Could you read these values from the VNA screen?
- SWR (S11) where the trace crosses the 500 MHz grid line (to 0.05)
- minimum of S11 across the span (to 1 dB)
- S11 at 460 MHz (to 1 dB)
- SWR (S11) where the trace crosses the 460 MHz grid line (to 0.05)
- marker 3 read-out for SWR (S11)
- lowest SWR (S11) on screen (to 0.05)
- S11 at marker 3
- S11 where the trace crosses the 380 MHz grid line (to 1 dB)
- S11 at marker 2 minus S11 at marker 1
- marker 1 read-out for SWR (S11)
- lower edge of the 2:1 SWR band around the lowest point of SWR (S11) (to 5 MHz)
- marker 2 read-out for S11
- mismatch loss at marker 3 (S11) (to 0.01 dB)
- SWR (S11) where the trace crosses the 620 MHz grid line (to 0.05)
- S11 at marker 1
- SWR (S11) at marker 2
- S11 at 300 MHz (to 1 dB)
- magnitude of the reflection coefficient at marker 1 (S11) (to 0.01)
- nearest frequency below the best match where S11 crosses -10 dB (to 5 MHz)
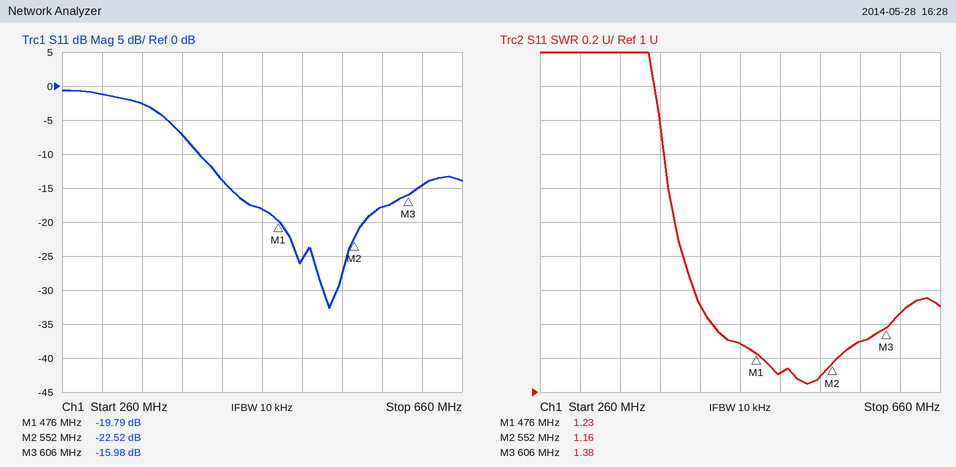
1.10
-33 dB
-18 dB
1.30
1.38
1.05
-15.98 dB
-7 dB
-2.73 dB
1.23
395 MHz
-22.52 dB
0.11 dB
1.45
-19.79 dB
1.16
-1 dB
0.10
395 MHz
